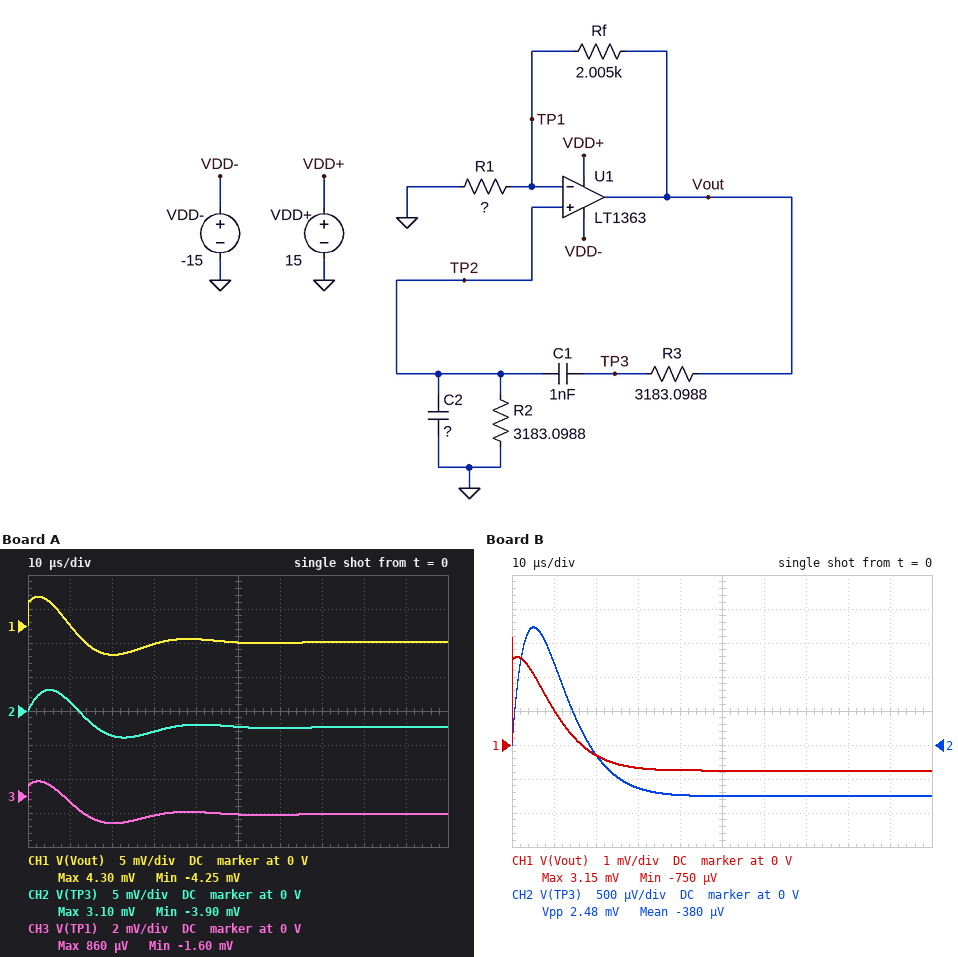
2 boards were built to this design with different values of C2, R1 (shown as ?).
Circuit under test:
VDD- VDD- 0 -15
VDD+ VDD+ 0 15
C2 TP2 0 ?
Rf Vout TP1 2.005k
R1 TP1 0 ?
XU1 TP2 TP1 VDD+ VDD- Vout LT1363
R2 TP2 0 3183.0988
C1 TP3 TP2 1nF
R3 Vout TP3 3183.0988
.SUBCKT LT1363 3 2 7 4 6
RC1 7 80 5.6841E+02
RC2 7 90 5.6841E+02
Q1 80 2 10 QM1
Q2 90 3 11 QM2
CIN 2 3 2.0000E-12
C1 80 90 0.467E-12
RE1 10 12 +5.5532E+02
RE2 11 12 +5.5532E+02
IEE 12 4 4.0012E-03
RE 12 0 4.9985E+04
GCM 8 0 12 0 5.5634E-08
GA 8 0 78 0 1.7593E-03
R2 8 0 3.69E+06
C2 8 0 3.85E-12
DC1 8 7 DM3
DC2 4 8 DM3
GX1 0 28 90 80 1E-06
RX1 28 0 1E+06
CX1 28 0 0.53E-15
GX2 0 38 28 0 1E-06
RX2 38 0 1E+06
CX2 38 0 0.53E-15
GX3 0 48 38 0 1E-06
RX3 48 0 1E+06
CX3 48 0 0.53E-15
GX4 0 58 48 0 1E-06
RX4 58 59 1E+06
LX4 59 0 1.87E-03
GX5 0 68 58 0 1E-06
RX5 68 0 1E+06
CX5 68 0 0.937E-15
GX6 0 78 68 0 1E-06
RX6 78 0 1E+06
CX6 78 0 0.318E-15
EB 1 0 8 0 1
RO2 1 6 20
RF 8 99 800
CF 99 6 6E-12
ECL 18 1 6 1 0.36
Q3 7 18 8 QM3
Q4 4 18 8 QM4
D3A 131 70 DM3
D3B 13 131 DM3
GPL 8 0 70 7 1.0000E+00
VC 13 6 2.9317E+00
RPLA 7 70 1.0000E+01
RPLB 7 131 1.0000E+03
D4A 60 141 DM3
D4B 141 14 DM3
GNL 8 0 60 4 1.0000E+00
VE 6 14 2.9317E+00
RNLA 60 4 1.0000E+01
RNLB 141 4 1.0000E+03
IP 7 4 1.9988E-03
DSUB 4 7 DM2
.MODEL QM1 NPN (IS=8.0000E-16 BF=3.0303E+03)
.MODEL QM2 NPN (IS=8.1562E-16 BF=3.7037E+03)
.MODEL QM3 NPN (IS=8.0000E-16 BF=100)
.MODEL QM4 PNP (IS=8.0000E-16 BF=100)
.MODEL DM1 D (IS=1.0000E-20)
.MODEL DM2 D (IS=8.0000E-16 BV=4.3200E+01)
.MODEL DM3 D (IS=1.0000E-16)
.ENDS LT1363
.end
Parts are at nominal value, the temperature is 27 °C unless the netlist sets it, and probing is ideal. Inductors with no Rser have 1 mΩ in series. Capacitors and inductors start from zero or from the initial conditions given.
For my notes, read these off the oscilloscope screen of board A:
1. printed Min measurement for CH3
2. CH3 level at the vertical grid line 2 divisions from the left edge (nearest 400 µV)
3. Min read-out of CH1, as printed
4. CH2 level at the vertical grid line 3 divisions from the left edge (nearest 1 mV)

-1.60 mV
-1.6 mV
-4.25 mV
-3 mV
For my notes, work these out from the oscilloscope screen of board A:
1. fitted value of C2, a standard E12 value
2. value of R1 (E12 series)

2.7 nF
820 Ω
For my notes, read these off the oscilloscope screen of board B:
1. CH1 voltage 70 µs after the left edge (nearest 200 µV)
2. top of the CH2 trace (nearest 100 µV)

-800 µV
1.7 mV
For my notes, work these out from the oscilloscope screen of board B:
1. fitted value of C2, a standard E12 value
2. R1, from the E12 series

3.3 nF
2.2 kΩ
